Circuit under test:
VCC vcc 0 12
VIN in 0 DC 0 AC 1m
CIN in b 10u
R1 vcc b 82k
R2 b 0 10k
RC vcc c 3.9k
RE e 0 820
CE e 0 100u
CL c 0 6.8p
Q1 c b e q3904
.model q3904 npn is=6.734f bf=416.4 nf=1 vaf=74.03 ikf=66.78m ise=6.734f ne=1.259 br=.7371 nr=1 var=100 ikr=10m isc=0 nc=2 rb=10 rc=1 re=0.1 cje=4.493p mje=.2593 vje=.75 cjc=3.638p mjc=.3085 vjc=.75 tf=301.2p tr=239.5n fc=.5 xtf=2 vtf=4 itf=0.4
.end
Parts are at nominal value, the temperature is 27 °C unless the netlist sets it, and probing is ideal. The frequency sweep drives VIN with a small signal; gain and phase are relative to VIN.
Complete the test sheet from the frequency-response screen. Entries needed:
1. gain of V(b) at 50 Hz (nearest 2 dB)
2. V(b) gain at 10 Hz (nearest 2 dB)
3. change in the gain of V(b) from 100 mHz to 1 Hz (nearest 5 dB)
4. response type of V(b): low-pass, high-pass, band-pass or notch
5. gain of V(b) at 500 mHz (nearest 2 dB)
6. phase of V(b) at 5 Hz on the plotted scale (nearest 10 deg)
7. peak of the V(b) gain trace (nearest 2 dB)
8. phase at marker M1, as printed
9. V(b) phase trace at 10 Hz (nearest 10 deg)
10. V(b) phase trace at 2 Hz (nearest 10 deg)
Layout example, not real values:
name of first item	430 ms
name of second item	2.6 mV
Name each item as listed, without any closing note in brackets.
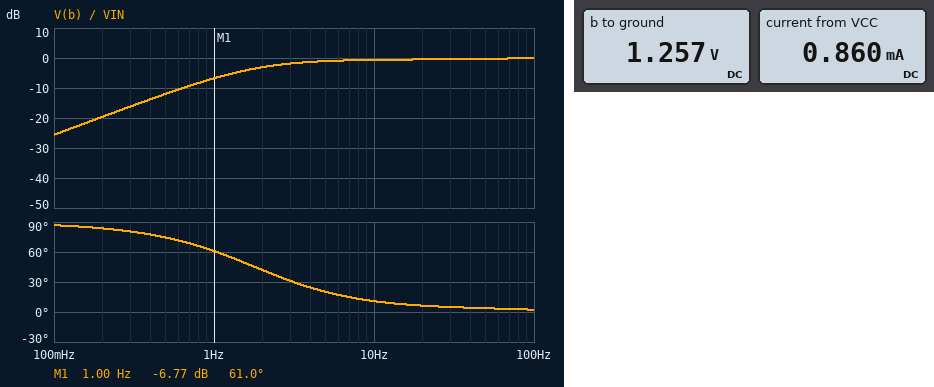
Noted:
gain of V(b) at 50 Hz	0 dB
V(b) gain at 10 Hz	0 dB
change in the gain of V(b) from 100 mHz to 1 Hz	20 dB
response type of V(b): low-pass, high-pass, band-pass or notch	high-pass
gain of V(b) at 500 mHz	-12 dB
phase of V(b) at 5 Hz on the plotted scale	20 deg
peak of the V(b) gain trace	0 dB
phase at marker M1, as printed	61.0 deg
V(b) phase trace at 10 Hz	10 deg
V(b) phase trace at 2 Hz	40 deg
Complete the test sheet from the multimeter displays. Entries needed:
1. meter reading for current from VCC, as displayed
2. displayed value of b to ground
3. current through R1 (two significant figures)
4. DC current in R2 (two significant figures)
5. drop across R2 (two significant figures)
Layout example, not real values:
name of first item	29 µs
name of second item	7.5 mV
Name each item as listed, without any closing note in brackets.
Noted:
meter reading for current from VCC, as displayed	0.860 mA
displayed value of b to ground	1.257 V
current through R1	130 µA
DC current in R2	130 µA
drop across R2	1.3 V
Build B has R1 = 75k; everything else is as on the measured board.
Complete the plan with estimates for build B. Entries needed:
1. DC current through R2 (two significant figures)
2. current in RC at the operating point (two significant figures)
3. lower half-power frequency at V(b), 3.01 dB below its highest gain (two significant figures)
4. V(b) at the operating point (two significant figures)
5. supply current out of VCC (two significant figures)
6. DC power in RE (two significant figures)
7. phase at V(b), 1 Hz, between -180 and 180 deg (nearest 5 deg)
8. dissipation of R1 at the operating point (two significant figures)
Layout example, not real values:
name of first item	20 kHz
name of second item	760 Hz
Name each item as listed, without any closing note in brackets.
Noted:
DC current through R2	140 µA
current in RC at the operating point	850 µA
lower half-power frequency at V(b), 3.01 dB below its highest gain	2.1 Hz
V(b) at the operating point	1.4 V
supply current out of VCC	990 µA
DC power in RE	600 µW
phase at V(b), 1 Hz, between -180 and 180 deg	60 deg
dissipation of R1 at the operating point	1.5 mW
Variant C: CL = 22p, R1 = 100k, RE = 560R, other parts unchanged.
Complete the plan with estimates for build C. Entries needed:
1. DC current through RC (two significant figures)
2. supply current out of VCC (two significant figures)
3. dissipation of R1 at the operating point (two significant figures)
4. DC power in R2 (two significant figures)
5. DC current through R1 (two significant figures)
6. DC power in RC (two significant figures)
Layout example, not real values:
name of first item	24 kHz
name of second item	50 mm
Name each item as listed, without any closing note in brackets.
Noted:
DC current through RC	690 µA
supply current out of VCC	800 µA
dissipation of R1 at the operating point	1.2 mW
DC power in R2	110 µW
DC current through R1	110 µA
DC power in RC	1.9 mW
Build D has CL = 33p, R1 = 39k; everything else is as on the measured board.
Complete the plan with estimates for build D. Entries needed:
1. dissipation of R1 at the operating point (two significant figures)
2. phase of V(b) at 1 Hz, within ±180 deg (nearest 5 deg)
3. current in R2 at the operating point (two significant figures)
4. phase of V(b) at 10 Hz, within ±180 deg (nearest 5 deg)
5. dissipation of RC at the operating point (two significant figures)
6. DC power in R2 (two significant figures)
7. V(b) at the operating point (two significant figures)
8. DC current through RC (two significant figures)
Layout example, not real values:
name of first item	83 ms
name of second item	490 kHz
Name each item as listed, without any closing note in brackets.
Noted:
dissipation of R1 at the operating point	2.4 mW
phase of V(b) at 1 Hz, within ±180 deg	65 deg
current in R2 at the operating point	230 µA
phase of V(b) at 10 Hz, within ±180 deg	10 deg
dissipation of RC at the operating point	16 mW
DC power in R2	550 µW
V(b) at the operating point	2.3 V
DC current through RC	2.0 mA
